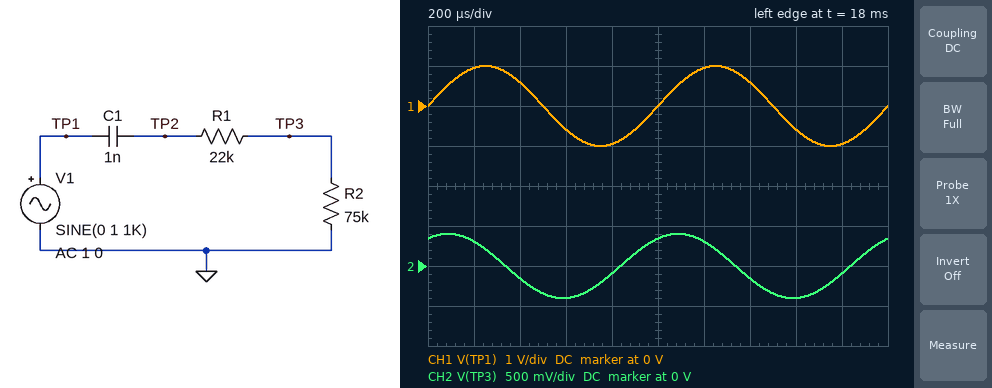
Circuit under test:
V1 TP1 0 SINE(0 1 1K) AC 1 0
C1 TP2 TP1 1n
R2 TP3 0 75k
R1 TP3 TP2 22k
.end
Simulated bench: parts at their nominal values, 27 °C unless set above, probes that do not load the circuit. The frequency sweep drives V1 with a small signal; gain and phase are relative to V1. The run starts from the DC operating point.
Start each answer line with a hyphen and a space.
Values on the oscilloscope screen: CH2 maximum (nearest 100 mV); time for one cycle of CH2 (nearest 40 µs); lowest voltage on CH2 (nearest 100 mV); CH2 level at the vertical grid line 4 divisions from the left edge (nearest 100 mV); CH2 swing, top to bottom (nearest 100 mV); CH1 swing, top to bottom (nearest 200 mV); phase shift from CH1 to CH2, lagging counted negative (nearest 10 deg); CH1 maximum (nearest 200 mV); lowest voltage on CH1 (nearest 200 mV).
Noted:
- 400 mV
- 1.00 ms
- -400 mV
- -100 mV
- 800 mV
- 2.0 V
- 60 deg
- 1.0 V
- -1.0 V
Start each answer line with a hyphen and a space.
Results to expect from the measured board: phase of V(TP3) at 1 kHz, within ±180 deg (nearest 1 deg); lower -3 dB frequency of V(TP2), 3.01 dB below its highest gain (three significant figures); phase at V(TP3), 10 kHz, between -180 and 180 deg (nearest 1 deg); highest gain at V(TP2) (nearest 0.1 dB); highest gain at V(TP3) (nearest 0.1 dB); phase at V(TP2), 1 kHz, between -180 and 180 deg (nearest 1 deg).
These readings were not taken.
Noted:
- 59 deg
- 1.64 kHz
- 9 deg
- 0 dB
- -2.2 dB
- 59 deg
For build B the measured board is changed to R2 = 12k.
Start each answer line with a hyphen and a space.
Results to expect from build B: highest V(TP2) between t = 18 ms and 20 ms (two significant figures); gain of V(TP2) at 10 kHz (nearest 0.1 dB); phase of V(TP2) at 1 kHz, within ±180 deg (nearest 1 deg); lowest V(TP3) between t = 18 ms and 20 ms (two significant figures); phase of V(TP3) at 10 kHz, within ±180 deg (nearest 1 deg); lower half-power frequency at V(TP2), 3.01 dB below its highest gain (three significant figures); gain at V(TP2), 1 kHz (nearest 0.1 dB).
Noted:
- 210 mV
- -0.9 dB
- 78 deg
- -74 mV
- 25 deg
- 4.68 kHz
- -13.6 dB
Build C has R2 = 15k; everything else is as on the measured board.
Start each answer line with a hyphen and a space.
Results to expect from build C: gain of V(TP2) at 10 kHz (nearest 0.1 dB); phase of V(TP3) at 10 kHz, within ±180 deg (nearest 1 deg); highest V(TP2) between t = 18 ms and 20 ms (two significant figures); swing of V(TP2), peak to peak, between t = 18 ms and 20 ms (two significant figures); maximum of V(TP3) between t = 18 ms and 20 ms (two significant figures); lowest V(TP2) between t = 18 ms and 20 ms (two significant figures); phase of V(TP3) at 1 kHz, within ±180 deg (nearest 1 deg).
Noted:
- -0.7 dB
- 23 deg
- 230 mV
- 450 mV
- 92 mV
- -230 mV
- 77 deg
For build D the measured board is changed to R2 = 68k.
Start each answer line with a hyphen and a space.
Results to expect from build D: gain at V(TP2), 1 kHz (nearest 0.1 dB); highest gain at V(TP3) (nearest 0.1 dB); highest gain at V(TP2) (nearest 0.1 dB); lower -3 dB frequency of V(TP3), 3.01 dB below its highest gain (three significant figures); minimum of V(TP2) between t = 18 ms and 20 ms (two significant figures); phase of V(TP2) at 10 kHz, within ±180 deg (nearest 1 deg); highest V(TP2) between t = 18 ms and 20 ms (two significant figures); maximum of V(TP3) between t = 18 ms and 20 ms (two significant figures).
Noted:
- -6.2 dB
- -2.4 dB
- 0 dB
- 1.77 kHz
- -490 mV
- 10 deg
- 490 mV
- 370 mV
